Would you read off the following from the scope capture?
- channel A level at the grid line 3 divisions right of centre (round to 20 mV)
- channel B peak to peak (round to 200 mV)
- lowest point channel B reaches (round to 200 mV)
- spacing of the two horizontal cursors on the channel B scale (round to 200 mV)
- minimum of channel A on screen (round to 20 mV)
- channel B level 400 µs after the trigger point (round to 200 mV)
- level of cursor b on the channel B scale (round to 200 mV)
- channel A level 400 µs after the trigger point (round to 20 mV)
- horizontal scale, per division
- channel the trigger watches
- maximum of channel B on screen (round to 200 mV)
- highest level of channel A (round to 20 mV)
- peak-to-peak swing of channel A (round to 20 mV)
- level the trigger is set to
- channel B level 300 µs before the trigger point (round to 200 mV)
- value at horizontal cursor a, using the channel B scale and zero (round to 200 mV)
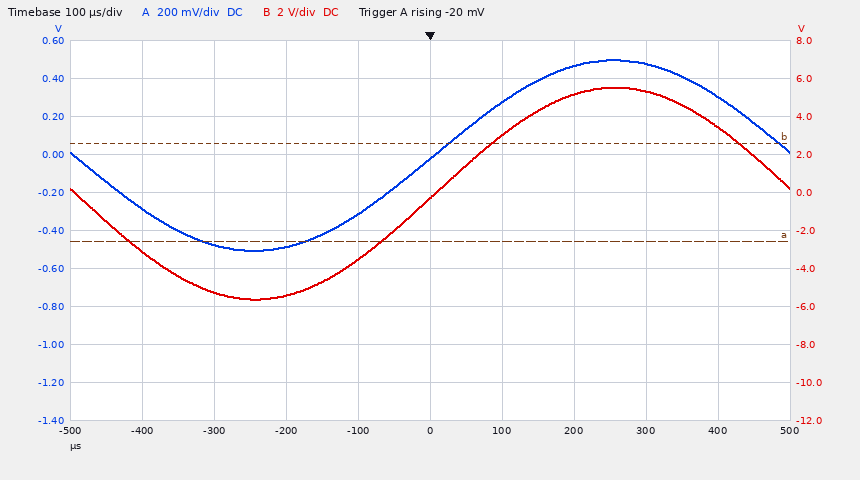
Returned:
480 mV
11.2 V
-5.6 V
5.2 V
-500 mV
3.4 V
2.6 V
300 mV
100 µs
channel A
5.6 V
500 mV
1.00 V
-20 mV
-5.2 V
-2.6 V
